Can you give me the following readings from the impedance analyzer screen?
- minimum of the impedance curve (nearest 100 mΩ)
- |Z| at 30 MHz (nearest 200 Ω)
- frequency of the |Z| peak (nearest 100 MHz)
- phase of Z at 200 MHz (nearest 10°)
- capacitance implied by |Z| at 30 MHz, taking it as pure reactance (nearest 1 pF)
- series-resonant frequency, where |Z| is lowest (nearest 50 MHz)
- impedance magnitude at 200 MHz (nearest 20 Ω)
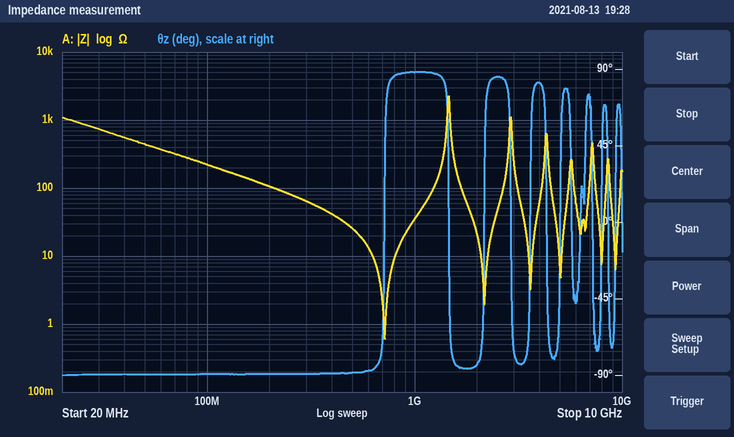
600 mΩ
800 Ω
1.5 GHz
-90°
7 pF
700 MHz
100 Ω
